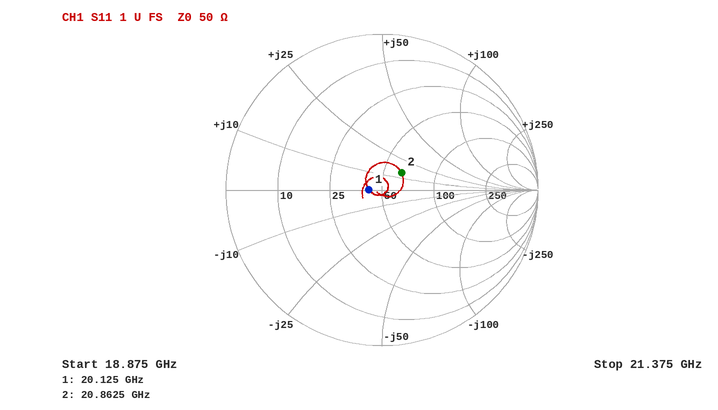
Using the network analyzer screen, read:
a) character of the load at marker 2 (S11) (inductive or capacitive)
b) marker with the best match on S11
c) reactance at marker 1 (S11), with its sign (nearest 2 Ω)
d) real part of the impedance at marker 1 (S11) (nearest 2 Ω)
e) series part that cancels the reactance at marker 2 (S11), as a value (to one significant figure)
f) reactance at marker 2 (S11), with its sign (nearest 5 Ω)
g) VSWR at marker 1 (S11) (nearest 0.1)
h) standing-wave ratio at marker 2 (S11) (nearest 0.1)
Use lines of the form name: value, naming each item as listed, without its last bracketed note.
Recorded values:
character of the load at marker 2 (S11): inductive
marker with the best match on S11: marker 1
reactance at marker 1 (S11), with its sign: 0 Ω
real part of the impedance at marker 1 (S11): 42 Ω
series part that cancels the reactance at marker 2 (S11), as a value: 500 fF
reactance at marker 2 (S11), with its sign: +15 Ω
VSWR at marker 1 (S11): 1.2
standing-wave ratio at marker 2 (S11): 1.4
